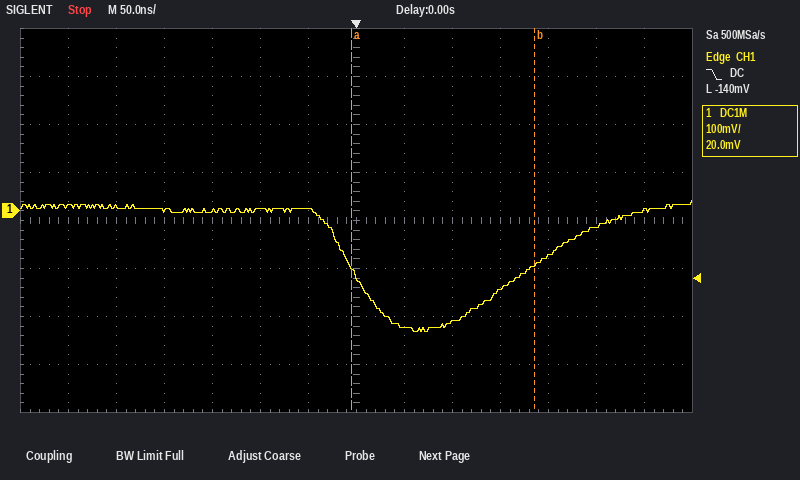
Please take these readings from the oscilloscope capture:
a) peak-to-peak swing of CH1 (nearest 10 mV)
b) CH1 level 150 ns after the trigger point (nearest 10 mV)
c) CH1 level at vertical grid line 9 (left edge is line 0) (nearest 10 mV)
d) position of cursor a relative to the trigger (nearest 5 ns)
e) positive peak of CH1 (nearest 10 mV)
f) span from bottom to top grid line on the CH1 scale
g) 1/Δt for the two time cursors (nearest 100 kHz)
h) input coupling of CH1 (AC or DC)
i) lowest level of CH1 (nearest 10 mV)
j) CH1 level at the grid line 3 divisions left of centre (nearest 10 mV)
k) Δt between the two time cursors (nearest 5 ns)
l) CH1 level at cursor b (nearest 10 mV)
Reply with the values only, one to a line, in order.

270 mV
-160 mV
-230 mV
-5 ns
20 mV
800 mV
5.3 MHz
DC
-250 mV
0 mV
190 ns
-110 mV
